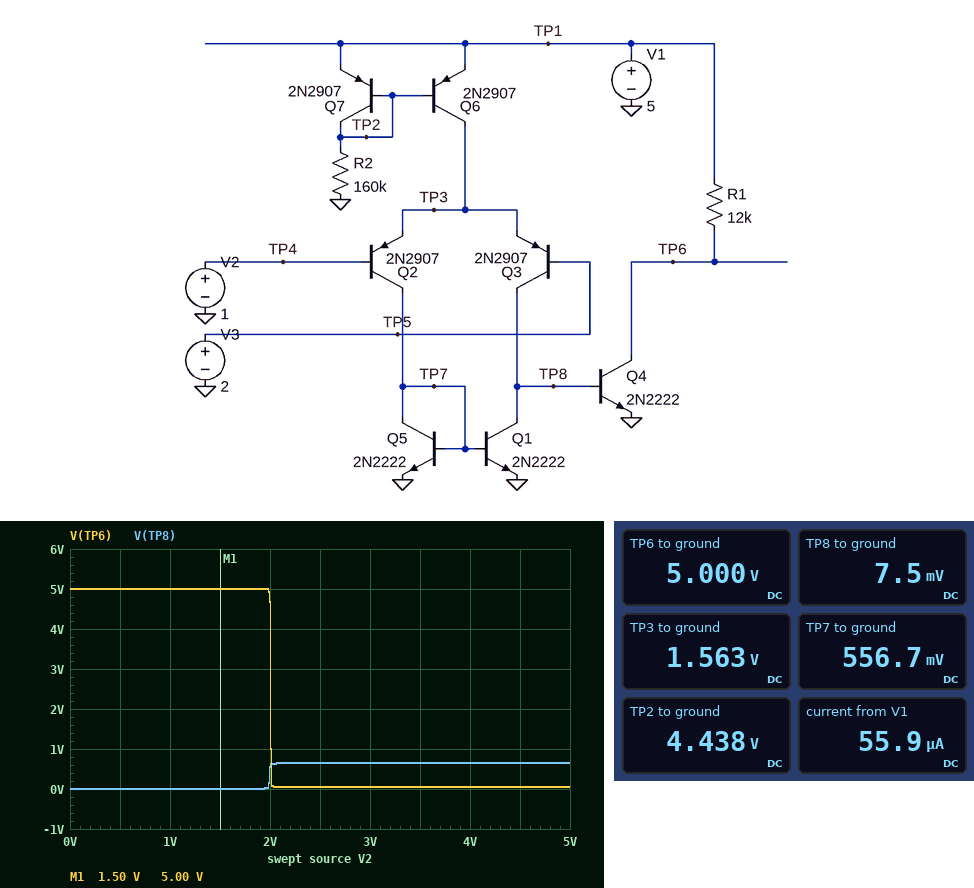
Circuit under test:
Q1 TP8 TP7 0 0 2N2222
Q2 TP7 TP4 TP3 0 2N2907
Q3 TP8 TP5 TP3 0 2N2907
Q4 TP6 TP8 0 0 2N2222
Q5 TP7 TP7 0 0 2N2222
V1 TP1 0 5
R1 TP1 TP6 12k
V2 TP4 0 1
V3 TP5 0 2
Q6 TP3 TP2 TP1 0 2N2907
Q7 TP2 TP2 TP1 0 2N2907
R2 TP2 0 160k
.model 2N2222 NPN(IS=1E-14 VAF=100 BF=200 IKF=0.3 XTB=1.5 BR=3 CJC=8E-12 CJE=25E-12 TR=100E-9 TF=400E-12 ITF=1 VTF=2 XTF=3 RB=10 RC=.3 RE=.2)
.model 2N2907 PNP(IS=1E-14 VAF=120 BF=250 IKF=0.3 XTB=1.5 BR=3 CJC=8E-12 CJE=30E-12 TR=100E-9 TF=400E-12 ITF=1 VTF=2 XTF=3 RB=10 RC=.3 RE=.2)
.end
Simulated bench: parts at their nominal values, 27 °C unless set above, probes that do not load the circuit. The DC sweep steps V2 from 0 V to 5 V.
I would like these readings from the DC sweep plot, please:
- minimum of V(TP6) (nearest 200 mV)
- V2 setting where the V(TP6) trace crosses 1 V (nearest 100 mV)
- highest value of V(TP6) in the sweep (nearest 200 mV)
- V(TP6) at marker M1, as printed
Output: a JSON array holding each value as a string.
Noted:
["0 V", "2.0 V", "5.0 V", "5.00 V"]
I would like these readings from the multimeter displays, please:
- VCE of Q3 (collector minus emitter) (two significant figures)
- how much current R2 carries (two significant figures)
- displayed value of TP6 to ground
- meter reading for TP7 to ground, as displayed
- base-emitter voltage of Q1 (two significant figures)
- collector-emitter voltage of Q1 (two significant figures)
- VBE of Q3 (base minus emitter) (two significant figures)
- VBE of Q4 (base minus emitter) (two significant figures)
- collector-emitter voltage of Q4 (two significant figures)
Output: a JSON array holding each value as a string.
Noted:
["-1.6 V", "28 µA", "5.000 V", "556.7 mV", "560 mV", "7.5 mV", "440 mV", "7.5 mV", "5.0 V"]
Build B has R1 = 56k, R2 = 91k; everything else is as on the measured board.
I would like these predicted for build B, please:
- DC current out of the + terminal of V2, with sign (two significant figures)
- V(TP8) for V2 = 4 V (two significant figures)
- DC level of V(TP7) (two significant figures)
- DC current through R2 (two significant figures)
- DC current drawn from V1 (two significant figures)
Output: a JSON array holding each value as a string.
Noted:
["-200 nA", "620 mV", "570 mV", "49 µA", "98 µA"]
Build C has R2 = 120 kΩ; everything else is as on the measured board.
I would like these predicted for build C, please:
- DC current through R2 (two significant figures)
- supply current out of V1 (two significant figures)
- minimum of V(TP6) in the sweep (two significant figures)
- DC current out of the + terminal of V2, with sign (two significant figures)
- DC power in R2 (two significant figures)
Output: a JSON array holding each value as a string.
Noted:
["37 µA", "74 µA", "44 mV", "-150 nA", "160 µW"]
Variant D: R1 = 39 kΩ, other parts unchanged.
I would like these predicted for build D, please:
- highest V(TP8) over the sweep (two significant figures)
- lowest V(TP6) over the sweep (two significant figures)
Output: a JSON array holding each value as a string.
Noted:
["620 mV", "28 mV"]
